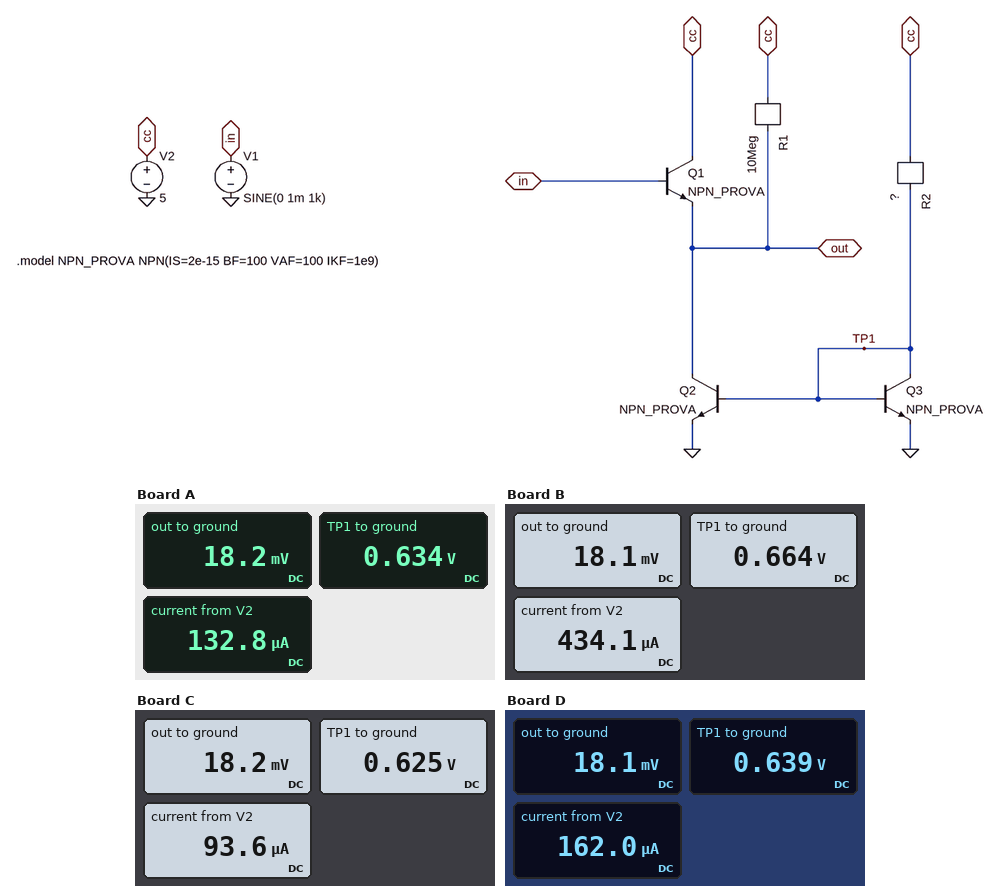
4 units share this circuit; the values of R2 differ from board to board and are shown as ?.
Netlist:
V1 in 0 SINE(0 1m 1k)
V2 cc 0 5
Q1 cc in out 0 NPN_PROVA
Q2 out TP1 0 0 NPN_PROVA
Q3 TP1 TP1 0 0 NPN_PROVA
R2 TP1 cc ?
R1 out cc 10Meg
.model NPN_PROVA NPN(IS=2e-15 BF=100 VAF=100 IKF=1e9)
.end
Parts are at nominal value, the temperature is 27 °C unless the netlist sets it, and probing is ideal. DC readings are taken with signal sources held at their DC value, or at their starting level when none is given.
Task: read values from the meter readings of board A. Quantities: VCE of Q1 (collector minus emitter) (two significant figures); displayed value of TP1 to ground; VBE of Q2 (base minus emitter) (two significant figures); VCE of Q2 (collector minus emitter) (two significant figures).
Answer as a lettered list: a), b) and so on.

a) 5.0 V
b) 0.634 V
c) 630 mV
d) 18 mV
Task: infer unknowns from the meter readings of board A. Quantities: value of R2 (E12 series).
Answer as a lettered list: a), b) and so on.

a) 33 kΩ
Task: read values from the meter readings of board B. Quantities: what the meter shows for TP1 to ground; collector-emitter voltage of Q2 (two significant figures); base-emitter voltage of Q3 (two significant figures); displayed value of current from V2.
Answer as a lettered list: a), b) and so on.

a) 0.664 V
b) 18 mV
c) 660 mV
d) 434.1 µA
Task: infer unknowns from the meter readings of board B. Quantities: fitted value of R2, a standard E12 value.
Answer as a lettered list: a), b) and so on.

a) 10 kΩ
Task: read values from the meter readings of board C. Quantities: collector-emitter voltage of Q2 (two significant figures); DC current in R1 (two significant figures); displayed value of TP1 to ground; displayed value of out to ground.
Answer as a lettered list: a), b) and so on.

a) 18 mV
b) 500 nA
c) 0.625 V
d) 18.2 mV
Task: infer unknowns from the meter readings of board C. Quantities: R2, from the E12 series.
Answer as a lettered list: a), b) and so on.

a) 47 kΩ
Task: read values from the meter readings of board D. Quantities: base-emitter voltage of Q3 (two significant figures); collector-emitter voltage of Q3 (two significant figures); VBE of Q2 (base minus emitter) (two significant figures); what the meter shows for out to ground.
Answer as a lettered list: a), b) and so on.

a) 640 mV
b) 640 mV
c) 640 mV
d) 18.1 mV
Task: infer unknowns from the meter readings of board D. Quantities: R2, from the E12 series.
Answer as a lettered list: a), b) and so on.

a) 27 kΩ
